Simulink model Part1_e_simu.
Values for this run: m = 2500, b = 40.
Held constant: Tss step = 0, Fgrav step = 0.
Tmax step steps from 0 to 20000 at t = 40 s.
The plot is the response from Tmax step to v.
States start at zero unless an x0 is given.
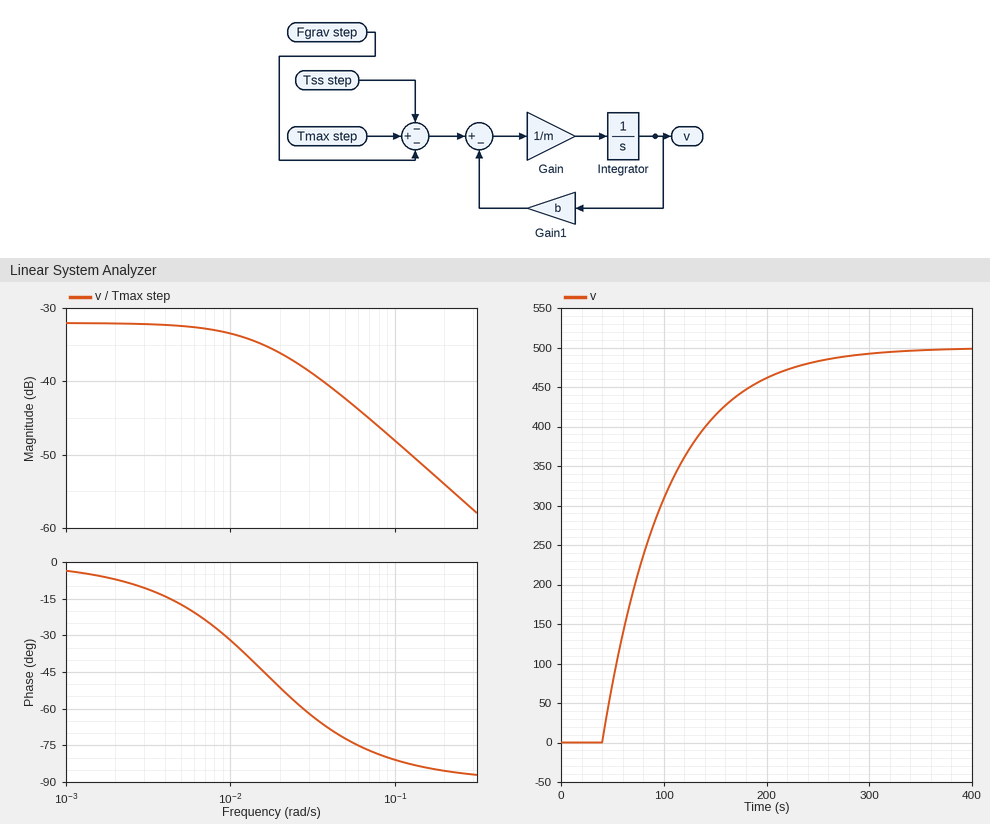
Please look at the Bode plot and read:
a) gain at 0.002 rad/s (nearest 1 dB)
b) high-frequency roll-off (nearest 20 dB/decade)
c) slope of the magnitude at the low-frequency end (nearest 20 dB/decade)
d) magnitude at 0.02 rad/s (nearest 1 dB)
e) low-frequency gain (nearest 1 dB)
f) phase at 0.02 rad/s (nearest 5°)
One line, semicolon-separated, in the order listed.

-32 dB; -20 dB/decade; 0 dB/decade; -36 dB; -32 dB; -50°
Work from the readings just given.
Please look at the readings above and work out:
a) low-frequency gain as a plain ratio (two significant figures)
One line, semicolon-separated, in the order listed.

0.025
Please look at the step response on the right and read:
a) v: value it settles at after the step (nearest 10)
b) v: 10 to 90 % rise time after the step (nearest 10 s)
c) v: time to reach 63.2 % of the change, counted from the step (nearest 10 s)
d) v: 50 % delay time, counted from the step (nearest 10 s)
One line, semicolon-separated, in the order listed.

500; 140 s; 60 s; 40 s
